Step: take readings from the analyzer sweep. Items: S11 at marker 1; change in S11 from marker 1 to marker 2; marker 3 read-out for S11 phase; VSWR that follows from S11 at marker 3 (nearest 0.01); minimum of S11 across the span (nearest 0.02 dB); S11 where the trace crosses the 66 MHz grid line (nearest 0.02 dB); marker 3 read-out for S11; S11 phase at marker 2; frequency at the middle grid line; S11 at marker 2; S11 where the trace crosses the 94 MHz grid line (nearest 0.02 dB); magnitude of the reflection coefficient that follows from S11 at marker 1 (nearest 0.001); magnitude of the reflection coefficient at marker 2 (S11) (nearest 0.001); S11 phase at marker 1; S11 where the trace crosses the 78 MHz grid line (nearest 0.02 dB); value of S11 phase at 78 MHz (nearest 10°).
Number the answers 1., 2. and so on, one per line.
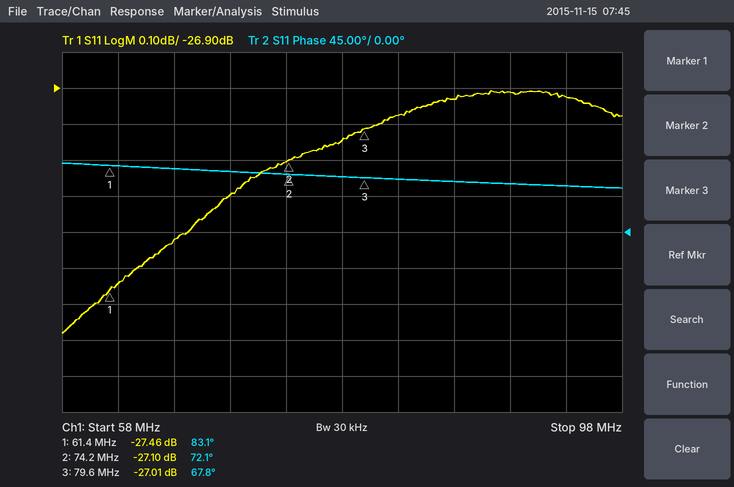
1. -27.46 dB
2. 0.36 dB
3. 67.8°
4. 1.09
5. -27.58 dB
6. -27.32 dB
7. -27.01 dB
8. 72.1°
9. 78 MHz
10. -27.10 dB
11. -26.92 dB
12. 0.042
13. 0.044
14. 83.1°
15. -27.04 dB
16. 70°
